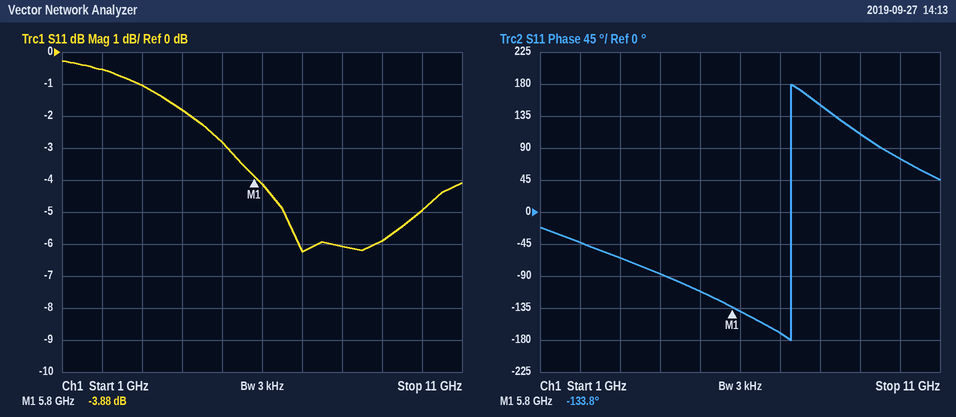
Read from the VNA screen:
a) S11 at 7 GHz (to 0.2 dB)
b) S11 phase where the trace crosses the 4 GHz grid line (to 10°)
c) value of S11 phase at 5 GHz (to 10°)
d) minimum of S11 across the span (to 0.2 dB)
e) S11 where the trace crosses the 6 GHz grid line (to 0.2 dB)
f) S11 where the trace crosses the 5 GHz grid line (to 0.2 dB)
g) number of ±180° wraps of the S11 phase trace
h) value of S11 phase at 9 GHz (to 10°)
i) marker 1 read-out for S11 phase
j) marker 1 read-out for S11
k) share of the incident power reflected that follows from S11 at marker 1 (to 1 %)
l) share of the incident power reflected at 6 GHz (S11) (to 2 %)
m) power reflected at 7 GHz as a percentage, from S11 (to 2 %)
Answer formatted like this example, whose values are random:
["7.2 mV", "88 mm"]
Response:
["-6.2 dB", "-90°", "-110°", "-6.2 dB", "-4.2 dB", "-2.8 dB", "1", "110°", "-133.8°", "-3.88 dB", "41 %", "38 %", "24 %"]
